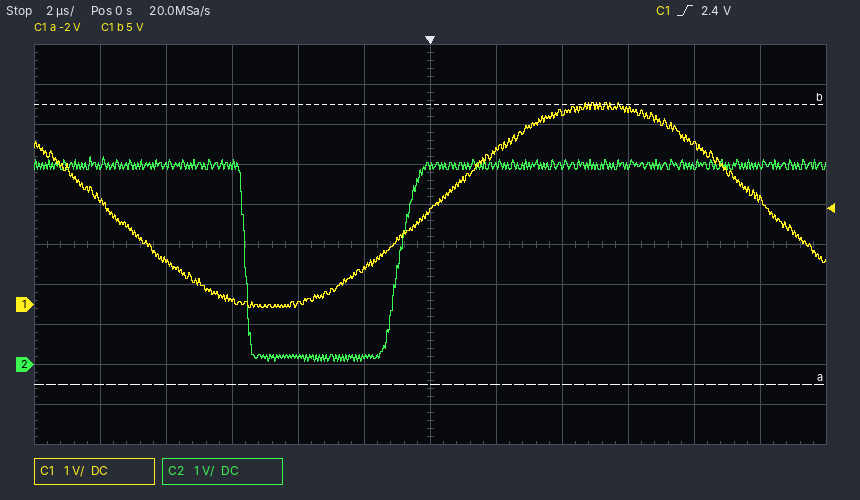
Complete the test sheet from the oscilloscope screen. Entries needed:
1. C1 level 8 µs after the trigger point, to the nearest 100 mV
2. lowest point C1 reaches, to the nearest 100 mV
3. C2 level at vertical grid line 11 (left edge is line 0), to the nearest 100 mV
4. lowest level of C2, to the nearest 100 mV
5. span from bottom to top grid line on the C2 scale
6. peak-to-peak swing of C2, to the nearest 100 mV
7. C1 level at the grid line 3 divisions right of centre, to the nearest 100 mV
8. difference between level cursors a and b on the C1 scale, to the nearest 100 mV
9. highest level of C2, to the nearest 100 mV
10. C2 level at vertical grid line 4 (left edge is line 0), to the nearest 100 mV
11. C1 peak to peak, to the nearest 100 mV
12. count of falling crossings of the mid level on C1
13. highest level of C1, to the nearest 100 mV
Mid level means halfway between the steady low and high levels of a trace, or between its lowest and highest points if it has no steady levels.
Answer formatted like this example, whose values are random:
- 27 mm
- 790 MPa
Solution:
- 4.0 V
- -100 mV
- 5.0 V
- 100 mV
- 10 V
- 5.1 V
- 4.9 V
- 7.0 V
- 5.2 V
- 200 mV
- 5.1 V
- 2
- 5.0 V
